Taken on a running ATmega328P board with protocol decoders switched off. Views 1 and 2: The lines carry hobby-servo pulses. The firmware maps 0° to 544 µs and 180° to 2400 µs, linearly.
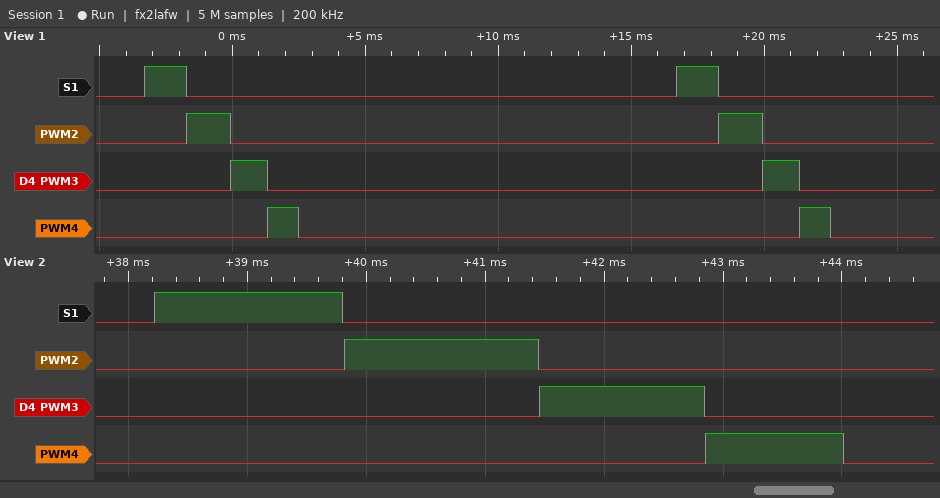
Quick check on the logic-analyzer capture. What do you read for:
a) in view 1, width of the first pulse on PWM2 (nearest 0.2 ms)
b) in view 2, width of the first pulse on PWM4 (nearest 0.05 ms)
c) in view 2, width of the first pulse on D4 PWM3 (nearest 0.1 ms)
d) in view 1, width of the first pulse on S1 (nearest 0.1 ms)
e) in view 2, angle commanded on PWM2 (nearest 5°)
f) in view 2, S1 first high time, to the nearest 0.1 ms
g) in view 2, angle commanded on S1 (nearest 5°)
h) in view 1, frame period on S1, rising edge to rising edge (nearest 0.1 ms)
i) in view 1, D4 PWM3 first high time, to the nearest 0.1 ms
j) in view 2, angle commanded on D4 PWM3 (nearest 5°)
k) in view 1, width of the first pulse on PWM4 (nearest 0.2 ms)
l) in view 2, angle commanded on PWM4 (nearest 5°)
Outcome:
1.6 ms
1.15 ms
1.4 ms
1.6 ms
105°
1.6 ms
100°
20.0 ms
1.4 ms
80°
1.2 ms
60°
